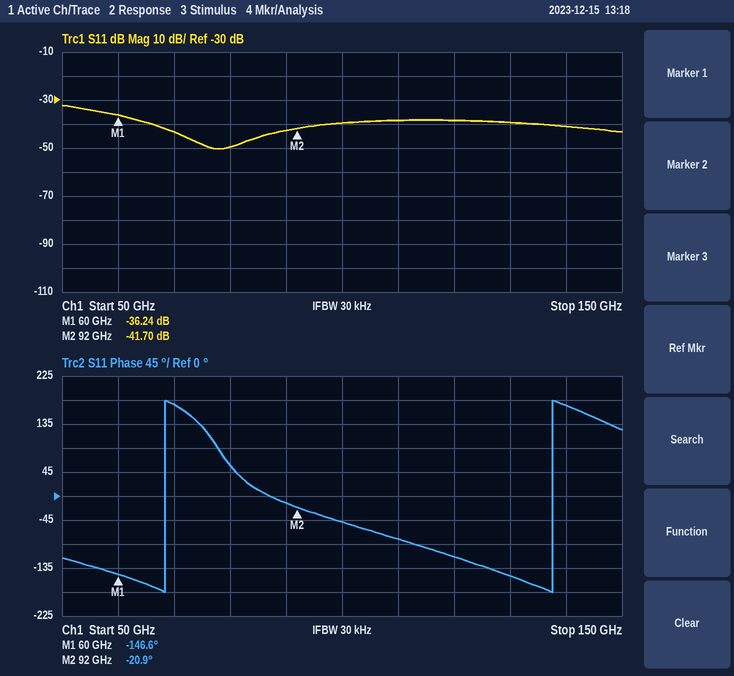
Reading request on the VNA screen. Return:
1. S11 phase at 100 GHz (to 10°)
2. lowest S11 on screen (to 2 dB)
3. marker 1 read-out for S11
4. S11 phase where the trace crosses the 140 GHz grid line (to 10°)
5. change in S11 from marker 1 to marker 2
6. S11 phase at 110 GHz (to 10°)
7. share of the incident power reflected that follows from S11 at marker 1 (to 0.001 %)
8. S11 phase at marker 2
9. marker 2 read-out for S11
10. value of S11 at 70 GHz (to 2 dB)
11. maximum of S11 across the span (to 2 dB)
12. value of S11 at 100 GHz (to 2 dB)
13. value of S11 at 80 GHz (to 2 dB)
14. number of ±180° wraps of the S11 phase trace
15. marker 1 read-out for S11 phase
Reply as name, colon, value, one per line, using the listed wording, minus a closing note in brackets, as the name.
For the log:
S11 phase at 100 GHz: -50°
lowest S11 on screen: -50 dB
marker 1 read-out for S11: -36.24 dB
S11 phase where the trace crosses the 140 GHz grid line: 170°
change in S11 from marker 1 to marker 2: -5.46 dB
S11 phase at 110 GHz: -80°
share of the incident power reflected that follows from S11 at marker 1: 0.024 %
S11 phase at marker 2: -20.9°
marker 2 read-out for S11: -41.70 dB
value of S11 at 70 GHz: -44 dB
maximum of S11 across the span: -32 dB
value of S11 at 100 GHz: -40 dB
value of S11 at 80 GHz: -50 dB
number of ±180° wraps of the S11 phase trace: 2
marker 1 read-out for S11 phase: -146.6°
